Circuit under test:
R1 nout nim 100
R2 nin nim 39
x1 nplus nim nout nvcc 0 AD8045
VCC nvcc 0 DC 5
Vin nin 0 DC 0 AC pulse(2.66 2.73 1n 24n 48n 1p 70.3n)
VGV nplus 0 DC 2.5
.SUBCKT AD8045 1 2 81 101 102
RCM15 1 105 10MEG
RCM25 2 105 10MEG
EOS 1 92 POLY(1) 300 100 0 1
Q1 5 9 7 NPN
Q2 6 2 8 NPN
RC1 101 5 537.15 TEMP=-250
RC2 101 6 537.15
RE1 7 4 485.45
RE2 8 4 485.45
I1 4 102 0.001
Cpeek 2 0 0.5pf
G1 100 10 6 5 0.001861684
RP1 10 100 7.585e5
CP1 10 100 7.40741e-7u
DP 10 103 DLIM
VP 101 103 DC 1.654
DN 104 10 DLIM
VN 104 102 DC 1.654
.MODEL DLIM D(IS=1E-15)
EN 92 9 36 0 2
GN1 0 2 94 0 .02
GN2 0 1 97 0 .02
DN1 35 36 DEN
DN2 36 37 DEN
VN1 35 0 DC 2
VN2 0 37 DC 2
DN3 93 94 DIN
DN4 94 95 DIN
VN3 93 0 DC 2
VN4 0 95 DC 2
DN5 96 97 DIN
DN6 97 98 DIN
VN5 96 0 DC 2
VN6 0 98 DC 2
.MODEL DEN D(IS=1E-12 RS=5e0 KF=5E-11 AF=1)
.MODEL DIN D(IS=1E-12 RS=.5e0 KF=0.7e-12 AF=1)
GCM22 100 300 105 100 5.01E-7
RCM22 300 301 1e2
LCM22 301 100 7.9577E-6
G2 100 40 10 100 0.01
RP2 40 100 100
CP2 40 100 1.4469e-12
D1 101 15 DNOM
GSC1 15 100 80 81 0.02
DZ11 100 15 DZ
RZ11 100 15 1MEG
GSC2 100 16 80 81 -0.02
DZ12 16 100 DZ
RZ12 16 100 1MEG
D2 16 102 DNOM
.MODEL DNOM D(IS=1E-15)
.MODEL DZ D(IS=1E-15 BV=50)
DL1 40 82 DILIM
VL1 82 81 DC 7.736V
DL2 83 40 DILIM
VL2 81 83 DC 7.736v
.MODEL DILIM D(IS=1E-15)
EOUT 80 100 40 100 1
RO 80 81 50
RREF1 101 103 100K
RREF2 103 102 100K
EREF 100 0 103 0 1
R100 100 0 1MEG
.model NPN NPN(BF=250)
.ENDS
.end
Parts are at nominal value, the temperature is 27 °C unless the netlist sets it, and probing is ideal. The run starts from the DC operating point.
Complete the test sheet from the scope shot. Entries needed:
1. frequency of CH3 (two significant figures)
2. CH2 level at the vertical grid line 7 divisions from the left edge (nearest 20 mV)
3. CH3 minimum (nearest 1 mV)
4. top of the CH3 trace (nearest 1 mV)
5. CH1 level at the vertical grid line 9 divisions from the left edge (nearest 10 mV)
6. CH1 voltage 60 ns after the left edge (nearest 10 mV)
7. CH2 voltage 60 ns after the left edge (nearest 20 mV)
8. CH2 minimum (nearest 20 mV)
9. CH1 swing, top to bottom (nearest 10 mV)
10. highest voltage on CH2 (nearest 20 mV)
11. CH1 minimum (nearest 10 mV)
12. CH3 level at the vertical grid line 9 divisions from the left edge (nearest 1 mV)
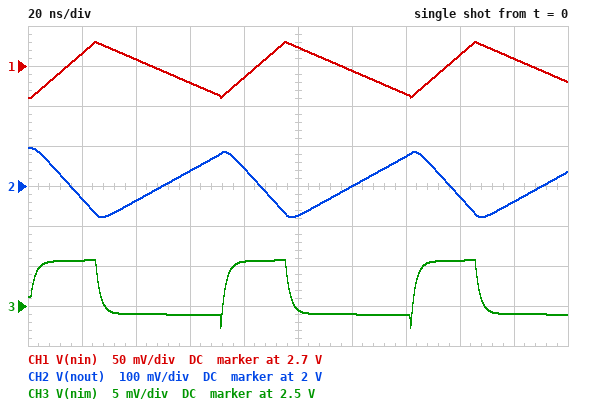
14 MHz
2.08 V
2.497 V
2.506 V
2.71 V
2.68 V
2.04 V
1.92 V
70 mV
2.10 V
2.66 V
2.499 V
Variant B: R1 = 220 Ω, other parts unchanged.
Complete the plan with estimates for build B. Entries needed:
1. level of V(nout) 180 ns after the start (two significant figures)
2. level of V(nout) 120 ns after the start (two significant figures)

1.3 V
1.4 V
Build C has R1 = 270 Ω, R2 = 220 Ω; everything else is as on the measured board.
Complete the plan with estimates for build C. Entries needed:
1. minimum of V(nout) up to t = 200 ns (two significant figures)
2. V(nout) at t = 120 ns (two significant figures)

2.2 V
2.3 V
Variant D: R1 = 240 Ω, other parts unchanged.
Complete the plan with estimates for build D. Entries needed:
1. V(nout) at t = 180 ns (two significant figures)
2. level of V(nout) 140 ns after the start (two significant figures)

1.3 V
1.5 V
